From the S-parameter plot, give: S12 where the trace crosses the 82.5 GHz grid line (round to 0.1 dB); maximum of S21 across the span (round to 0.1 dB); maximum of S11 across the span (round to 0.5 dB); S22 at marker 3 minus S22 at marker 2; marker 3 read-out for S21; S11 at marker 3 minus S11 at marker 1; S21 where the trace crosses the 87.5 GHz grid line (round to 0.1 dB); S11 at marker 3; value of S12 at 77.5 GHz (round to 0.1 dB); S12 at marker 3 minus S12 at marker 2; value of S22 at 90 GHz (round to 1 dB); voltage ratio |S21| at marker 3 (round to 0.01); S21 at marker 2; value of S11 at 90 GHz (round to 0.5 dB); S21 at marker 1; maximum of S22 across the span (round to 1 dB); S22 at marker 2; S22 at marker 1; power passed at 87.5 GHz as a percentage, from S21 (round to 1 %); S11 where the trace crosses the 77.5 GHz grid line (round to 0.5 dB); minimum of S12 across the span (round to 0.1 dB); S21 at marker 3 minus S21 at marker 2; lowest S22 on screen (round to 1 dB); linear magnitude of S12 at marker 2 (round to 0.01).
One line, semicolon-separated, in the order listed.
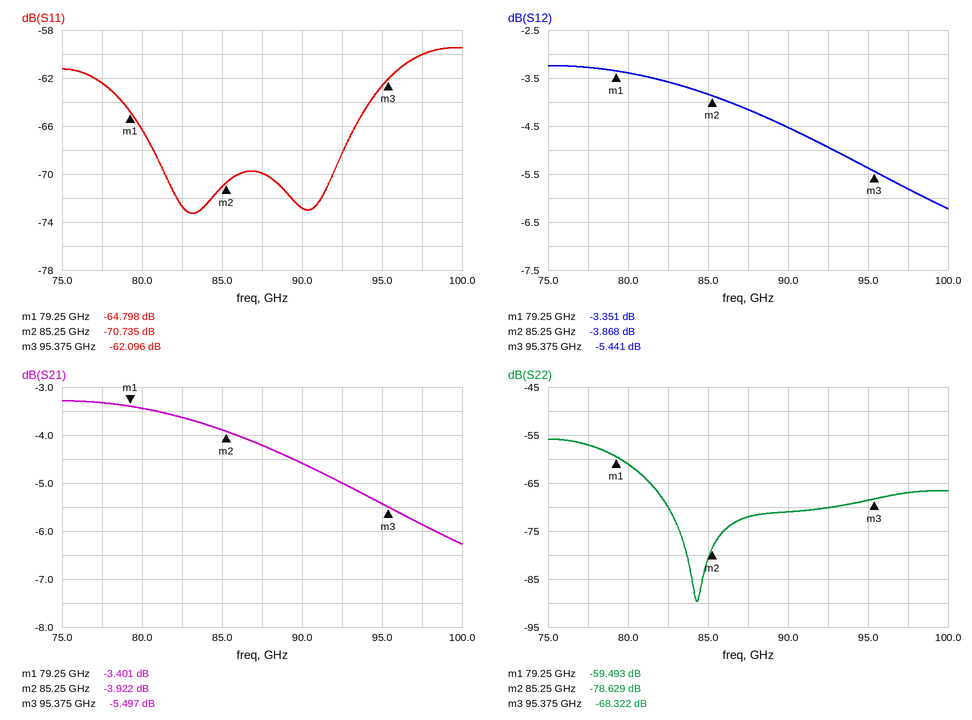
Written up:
-3.6 dB; -3.3 dB; -59.5 dB; 10.307 dB; -5.497 dB; 2.702 dB; -4.2 dB; -62.096 dB; -3.3 dB; -1.573 dB; -71 dB; 0.53; -3.922 dB; -73.0 dB; -3.401 dB; -56 dB; -78.629 dB; -59.493 dB; 38 %; -62.5 dB; -6.2 dB; -1.575 dB; -90 dB; 0.64
